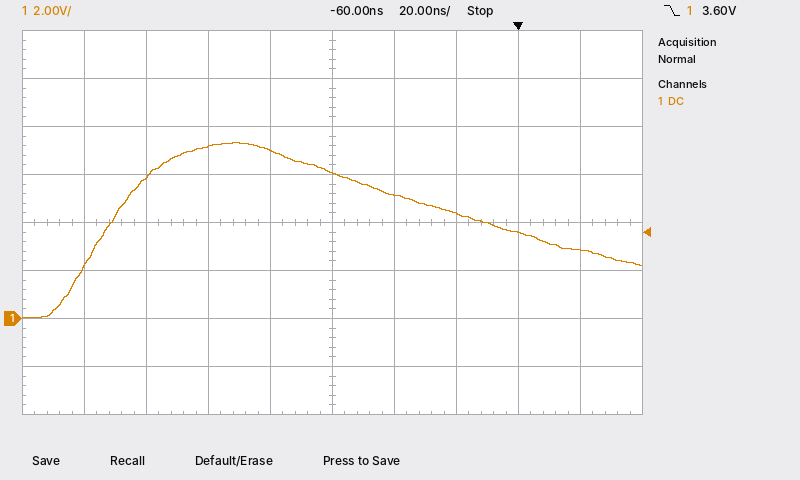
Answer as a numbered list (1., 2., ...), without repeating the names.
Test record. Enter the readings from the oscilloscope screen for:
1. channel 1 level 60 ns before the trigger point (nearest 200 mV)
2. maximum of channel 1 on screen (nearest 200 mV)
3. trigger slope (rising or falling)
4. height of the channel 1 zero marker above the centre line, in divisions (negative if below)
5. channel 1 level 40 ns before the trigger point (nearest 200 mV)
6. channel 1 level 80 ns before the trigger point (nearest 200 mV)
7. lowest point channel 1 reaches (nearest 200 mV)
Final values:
1. 6.0 V
2. 7.4 V
3. falling
4. -2.0 div
5. 5.2 V
6. 7.0 V
7. 0.0 V
